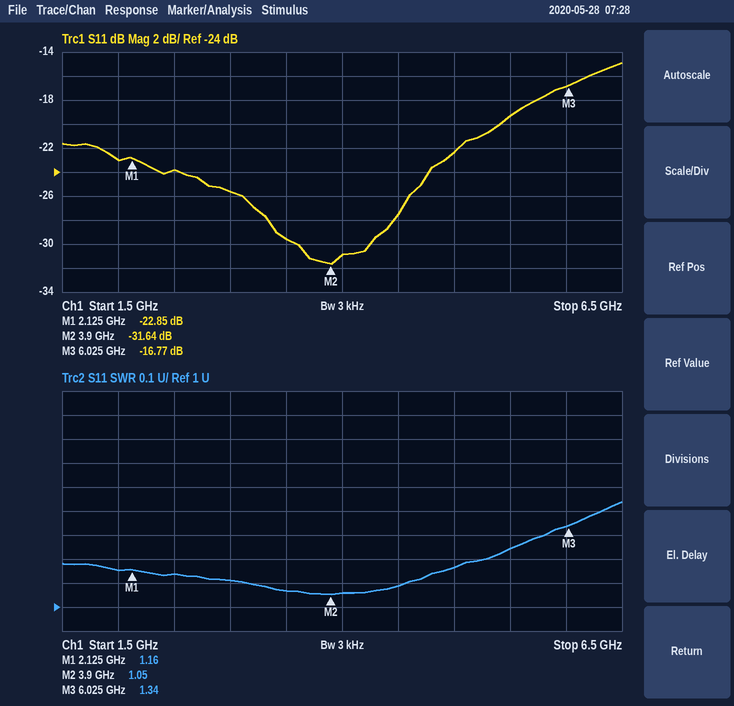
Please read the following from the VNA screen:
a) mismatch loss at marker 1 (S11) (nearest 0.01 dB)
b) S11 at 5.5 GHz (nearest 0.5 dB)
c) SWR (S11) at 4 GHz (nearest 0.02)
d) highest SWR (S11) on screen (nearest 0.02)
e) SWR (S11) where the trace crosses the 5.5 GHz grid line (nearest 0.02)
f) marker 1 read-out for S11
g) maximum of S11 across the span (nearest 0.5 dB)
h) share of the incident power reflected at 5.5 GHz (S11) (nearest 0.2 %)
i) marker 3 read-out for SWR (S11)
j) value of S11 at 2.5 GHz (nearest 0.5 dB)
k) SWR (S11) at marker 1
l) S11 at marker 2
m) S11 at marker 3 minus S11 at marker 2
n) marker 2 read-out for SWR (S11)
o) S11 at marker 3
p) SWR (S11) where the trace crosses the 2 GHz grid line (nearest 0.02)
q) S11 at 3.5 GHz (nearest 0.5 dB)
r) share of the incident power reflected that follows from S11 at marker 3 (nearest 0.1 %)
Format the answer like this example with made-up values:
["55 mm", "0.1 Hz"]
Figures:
["0.02 dB", "-19.5 dB", "1.06", "1.44", "1.24", "-22.85 dB", "-15.0 dB", "1.2 %", "1.34", "-24.0 dB", "1.16", "-31.64 dB", "14.87 dB", "1.05", "-16.77 dB", "1.16", "-29.5 dB", "2.1 %"]
